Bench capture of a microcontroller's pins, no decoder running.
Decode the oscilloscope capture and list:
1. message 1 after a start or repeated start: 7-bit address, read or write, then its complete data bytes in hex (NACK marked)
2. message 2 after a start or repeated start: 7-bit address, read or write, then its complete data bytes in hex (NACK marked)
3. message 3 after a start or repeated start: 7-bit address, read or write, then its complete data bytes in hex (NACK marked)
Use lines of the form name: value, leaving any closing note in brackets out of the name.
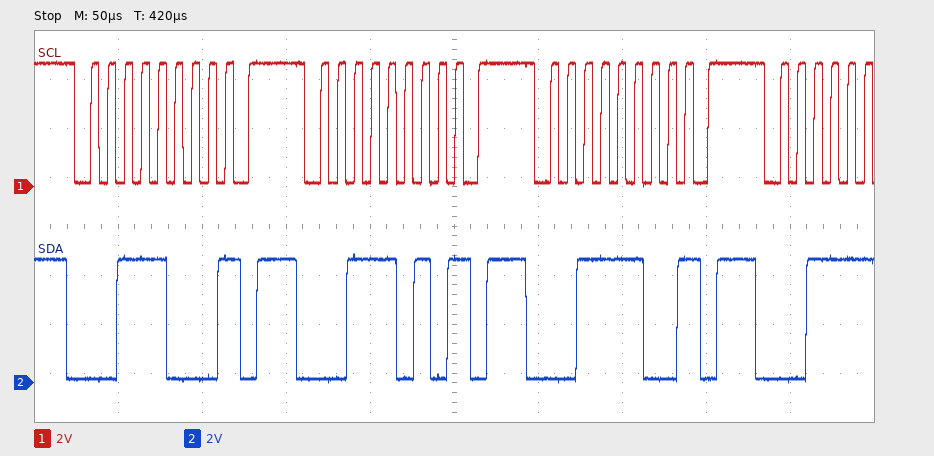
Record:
message 1 after a start or repeated start: 7-bit address, read or write, then its complete data bytes in hex: 0x1C write NACK
message 2 after a start or repeated start: 7-bit address, read or write, then its complete data bytes in hex: 0x1D write NACK
message 3 after a start or repeated start: 7-bit address, read or write, then its complete data bytes in hex: 0x1E write NACK
